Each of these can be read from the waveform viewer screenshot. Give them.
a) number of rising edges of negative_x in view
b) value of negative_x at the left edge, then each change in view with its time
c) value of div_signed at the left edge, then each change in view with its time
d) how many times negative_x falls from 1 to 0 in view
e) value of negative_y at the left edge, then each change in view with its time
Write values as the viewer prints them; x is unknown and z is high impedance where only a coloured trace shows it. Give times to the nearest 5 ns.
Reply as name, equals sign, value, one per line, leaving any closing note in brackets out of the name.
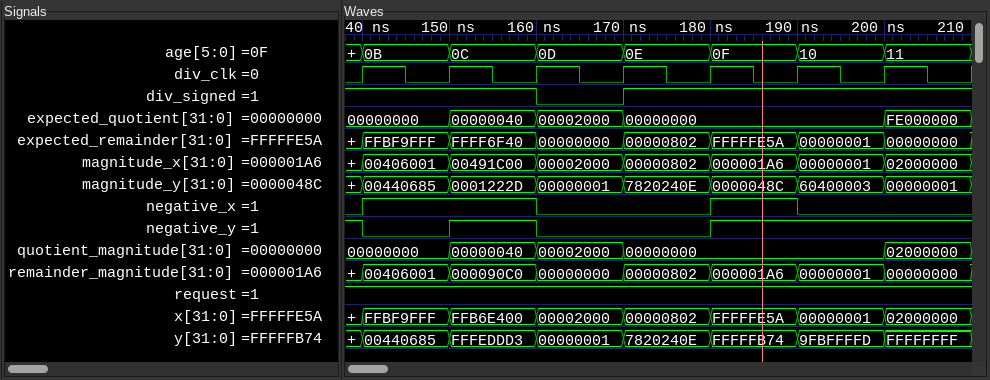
number of rising edges of negative_x in view = 2
value of negative_x at the left edge, then each change in view with its time = 0, 1 at 140 ns, 0 at 160 ns, 1 at 180 ns, 0 at 190 ns
value of div_signed at the left edge, then each change in view with its time = 1, 0 at 160 ns, 1 at 170 ns
how many times negative_x falls from 1 to 0 in view = 2
value of negative_y at the left edge, then each change in view with its time = 1, 0 at 140 ns, 1 at 150 ns, 0 at 160 ns, 1 at 180 ns
